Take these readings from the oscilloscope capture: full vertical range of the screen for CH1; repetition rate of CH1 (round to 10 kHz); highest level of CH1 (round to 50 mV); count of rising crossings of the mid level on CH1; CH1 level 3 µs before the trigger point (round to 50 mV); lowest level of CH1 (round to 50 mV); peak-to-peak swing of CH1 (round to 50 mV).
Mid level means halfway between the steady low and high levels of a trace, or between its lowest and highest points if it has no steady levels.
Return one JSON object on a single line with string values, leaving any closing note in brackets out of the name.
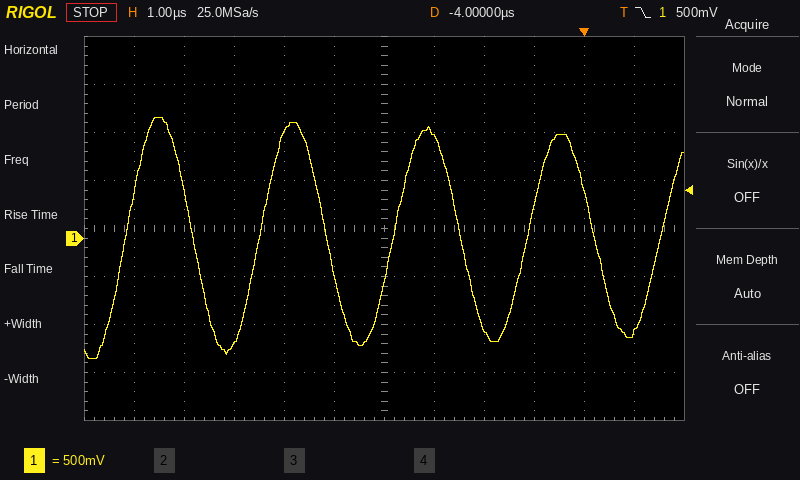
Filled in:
{"full vertical range of the screen for CH1": "4 V", "repetition rate of CH1": "370 kHz", "highest level of CH1": "1.25 V", "count of rising crossings of the mid level on CH1": "5", "CH1 level 3 µs before the trigger point": "1.05 V", "lowest level of CH1": "-1.25 V", "peak-to-peak swing of CH1": "2.50 V"}
